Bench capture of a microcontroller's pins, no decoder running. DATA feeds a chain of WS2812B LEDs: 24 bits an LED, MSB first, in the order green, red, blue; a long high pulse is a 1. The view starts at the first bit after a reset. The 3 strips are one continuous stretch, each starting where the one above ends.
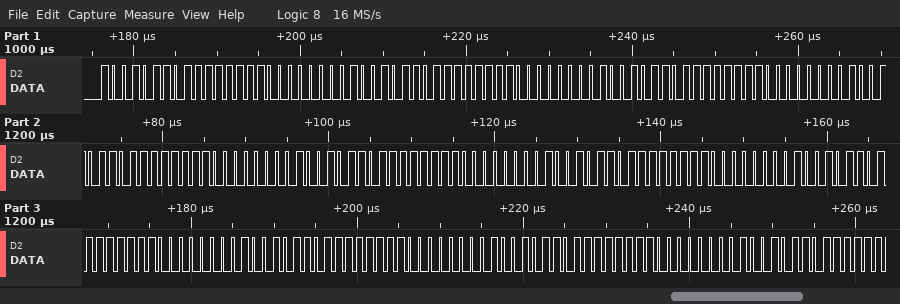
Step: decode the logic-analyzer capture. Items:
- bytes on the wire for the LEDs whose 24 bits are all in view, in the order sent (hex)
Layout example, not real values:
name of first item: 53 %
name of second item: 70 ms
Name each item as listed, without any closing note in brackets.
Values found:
bytes on the wire for the LEDs whose 24 bits are all in view, in the order sent: 96 FF 00 96 FF 00 96 FF 00 96 FF 00 96 FF 00 96 FF 00 96 FF 00 96 FF 00 96 FF 00
